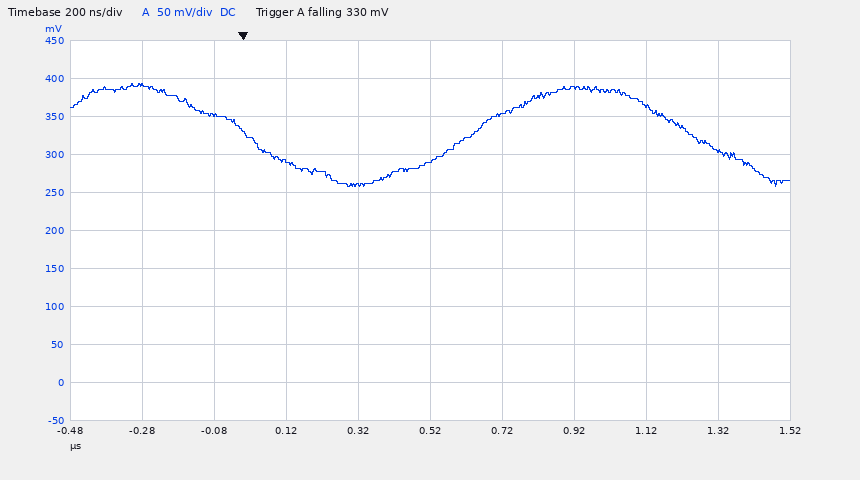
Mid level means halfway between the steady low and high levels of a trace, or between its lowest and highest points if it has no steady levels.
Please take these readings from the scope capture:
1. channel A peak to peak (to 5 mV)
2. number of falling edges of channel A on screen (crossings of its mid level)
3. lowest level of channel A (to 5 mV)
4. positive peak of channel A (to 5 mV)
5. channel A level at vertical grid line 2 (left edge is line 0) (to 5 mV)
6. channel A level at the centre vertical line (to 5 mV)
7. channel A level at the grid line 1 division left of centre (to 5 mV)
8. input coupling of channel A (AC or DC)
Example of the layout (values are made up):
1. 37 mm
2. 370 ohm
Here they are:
1. 135 mV
2. 2
3. 260 mV
4. 395 mV
5. 350 mV
6. 290 mV
7. 260 mV
8. DC
